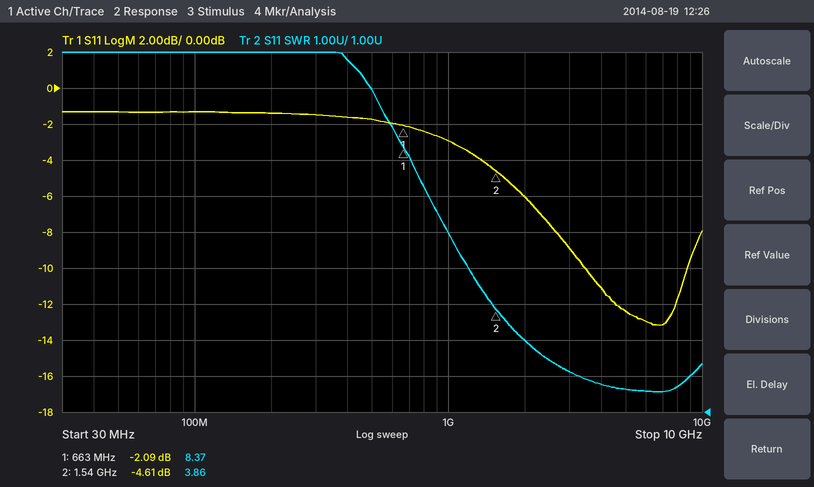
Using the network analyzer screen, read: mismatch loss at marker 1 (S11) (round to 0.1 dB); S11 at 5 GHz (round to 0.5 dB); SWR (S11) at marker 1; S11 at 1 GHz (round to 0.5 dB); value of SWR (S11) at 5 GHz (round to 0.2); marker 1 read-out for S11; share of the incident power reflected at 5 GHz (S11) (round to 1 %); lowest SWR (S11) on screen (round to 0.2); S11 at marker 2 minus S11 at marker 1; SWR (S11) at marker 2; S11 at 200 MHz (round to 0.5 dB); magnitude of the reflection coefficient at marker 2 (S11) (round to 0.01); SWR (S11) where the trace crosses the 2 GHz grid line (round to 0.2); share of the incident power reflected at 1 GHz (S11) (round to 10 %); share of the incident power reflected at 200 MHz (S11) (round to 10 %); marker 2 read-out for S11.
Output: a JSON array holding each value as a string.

["4.2 dB", "-12.5 dB", "8.37", "-3.0 dB", "1.6", "-2.09 dB", "6 %", "1.6", "-2.52 dB", "3.86", "-1.5 dB", "0.59", "3.0", "50 %", "70 %", "-4.61 dB"]
